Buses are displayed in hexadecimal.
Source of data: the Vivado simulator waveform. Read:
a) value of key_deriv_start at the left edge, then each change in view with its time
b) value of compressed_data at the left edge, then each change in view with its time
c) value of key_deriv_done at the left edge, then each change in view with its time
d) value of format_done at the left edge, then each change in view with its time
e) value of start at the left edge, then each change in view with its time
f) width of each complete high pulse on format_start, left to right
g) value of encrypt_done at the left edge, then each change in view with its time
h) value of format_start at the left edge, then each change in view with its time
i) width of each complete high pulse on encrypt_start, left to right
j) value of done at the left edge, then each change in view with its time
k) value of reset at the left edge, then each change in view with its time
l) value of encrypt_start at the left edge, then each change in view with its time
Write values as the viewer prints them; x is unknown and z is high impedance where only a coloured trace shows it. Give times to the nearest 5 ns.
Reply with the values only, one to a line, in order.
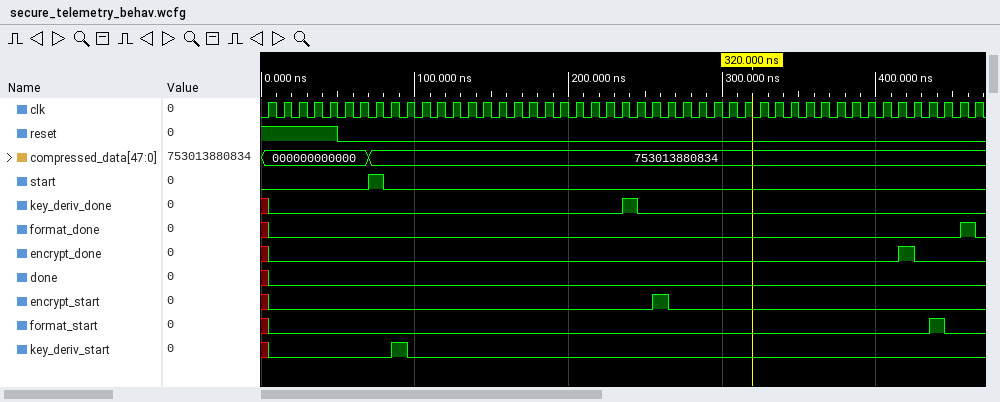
x, 0 at 5 ns, 1 at 85 ns, 0 at 95 ns
000000000000, 753013880834 at 70 ns
x, 0 at 5 ns, 1 at 235 ns, 0 at 245 ns
x, 0 at 5 ns, 1 at 455 ns, 0 at 465 ns
0, 1 at 70 ns, 0 at 80 ns
10 ns
x, 0 at 5 ns, 1 at 415 ns, 0 at 425 ns
x, 0 at 5 ns, 1 at 435 ns, 0 at 445 ns
10 ns
x, 0 at 5 ns
1, 0 at 50 ns
x, 0 at 5 ns, 1 at 255 ns, 0 at 265 ns
